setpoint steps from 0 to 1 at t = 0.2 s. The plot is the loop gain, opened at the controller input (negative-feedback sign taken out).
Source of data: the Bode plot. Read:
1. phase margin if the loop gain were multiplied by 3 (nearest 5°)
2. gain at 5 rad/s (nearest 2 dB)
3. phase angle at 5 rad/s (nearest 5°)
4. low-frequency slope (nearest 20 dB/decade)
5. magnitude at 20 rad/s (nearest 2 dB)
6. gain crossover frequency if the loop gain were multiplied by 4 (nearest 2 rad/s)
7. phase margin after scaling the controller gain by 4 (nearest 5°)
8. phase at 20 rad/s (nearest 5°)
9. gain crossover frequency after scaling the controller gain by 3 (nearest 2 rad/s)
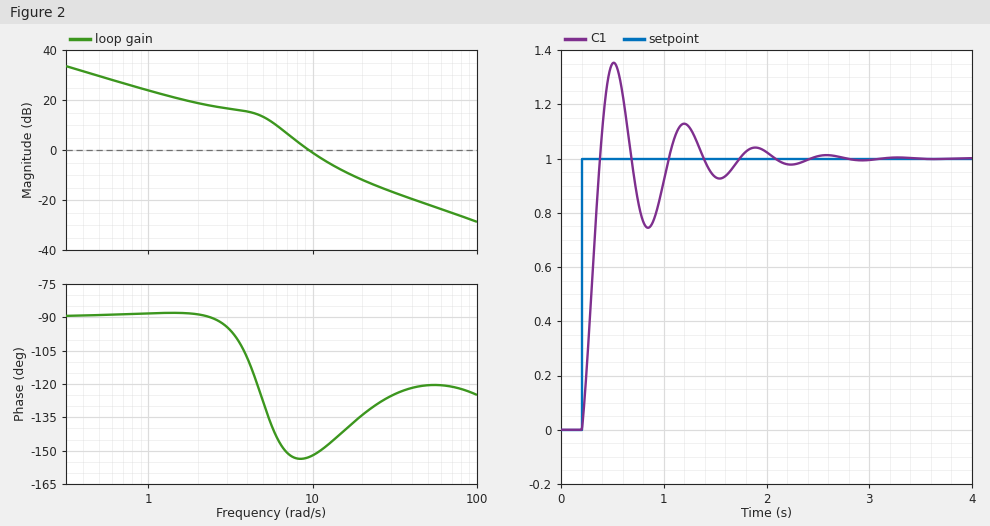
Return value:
40°
14 dB
-130°
-20 dB/decade
-12 dB
20 rad/s
45°
-135°
16 rad/s
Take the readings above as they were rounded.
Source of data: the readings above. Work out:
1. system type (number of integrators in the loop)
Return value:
1
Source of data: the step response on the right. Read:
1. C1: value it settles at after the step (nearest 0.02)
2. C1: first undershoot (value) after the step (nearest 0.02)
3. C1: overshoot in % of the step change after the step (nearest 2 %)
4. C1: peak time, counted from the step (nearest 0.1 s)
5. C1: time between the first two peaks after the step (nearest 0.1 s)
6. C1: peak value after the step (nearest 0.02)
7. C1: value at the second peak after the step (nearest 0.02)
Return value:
1.00
0.74
36 %
0.3 s
0.7 s
1.36
1.12
